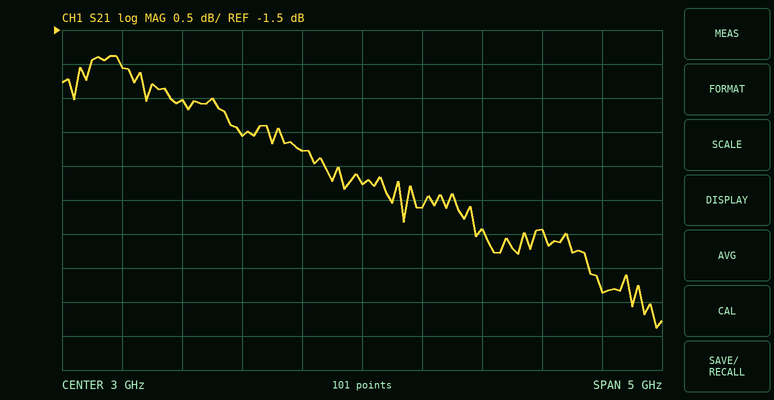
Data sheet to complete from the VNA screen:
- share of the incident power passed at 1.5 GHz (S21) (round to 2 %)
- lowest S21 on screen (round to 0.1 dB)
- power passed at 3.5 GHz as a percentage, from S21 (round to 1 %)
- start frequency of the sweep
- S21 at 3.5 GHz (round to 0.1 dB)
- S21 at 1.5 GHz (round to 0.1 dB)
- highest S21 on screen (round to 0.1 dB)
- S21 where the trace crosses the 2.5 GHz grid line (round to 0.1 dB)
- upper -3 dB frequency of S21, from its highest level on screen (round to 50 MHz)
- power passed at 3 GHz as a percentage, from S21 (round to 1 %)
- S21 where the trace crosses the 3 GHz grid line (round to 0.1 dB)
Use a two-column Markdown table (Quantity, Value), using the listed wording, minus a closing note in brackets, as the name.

| Quantity | Value |
|---|---|
| share of the incident power passed at 1.5 GHz (S21) | 56 % |
| lowest S21 on screen | -5.9 dB |
| power passed at 3.5 GHz as a percentage, from S21 | 39 % |
| start frequency of the sweep | 500 MHz |
| S21 at 3.5 GHz | -4.1 dB |
| S21 at 1.5 GHz | -2.5 dB |
| highest S21 on screen | -1.9 dB |
| S21 where the trace crosses the 2.5 GHz grid line | -3.3 dB |
| upper -3 dB frequency of S21, from its highest level on screen | 4.85 GHz |
| power passed at 3 GHz as a percentage, from S21 | 42 % |
| S21 where the trace crosses the 3 GHz grid line | -3.8 dB |
